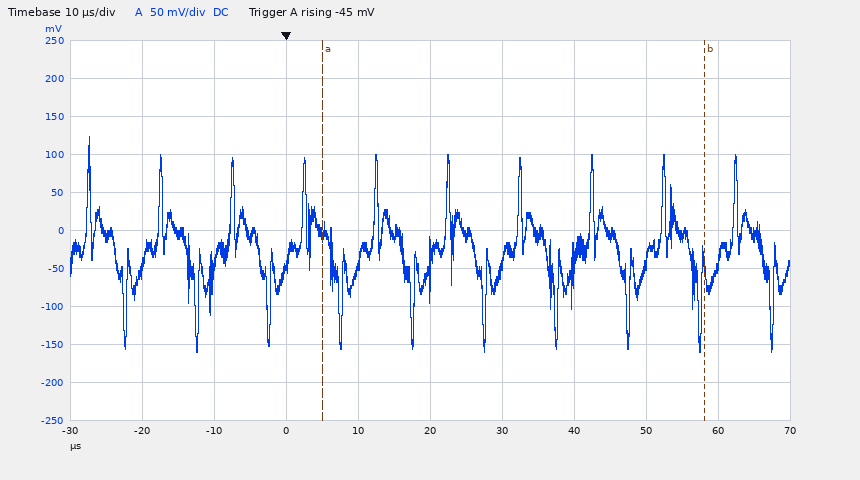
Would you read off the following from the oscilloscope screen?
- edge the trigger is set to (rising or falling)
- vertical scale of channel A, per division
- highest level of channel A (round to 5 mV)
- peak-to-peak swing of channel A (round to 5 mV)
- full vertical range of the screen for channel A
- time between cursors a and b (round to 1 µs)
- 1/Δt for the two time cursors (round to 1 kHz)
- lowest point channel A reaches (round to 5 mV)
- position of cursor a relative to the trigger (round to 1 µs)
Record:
rising
50 mV
125 mV
285 mV
500 mV
53 µs
19 kHz
-160 mV
+5 µs
